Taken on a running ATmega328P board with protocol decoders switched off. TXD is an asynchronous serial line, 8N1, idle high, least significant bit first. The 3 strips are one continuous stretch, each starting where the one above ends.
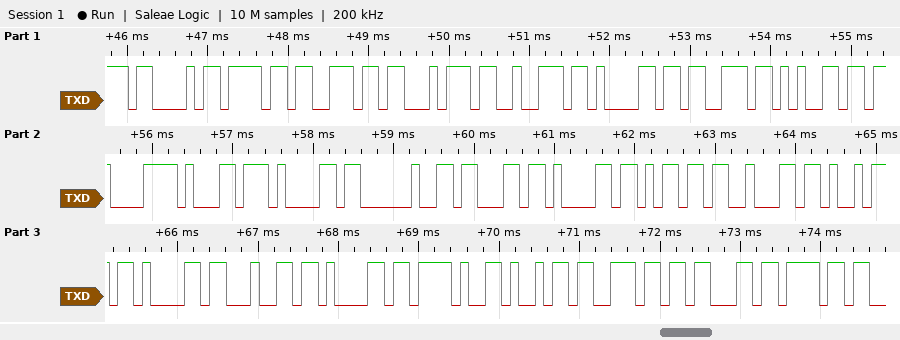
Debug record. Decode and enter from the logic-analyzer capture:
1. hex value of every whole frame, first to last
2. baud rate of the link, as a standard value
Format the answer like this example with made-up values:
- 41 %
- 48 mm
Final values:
- 43 6F 6E 74 72 61 73 65 C3 B1 61 20 63 61 6D 62 69 61 64 61 2F 69 6E 63 6F
- 9600 baud
